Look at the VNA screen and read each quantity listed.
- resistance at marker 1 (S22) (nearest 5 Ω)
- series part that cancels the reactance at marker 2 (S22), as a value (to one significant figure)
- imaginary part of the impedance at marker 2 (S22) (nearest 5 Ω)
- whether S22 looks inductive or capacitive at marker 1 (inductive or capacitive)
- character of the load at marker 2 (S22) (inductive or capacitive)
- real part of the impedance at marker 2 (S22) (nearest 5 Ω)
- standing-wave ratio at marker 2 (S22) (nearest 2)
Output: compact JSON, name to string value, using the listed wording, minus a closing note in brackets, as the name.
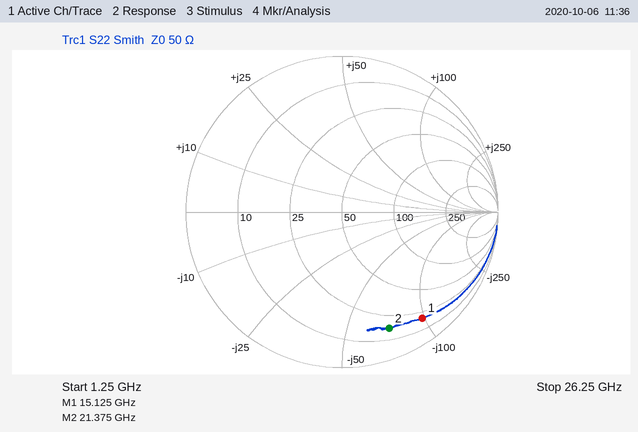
{"resistance at marker 1 (S22)": "20 Ω", "series part that cancels the reactance at marker 2 (S22), as a value": "500 pH", "imaginary part of the impedance at marker 2 (S22)": "-70 Ω", "whether S22 looks inductive or capacitive at marker 1": "capacitive", "character of the load at marker 2 (S22)": "capacitive", "real part of the impedance at marker 2 (S22)": "15 Ω", "standing-wave ratio at marker 2 (S22)": "10"}
